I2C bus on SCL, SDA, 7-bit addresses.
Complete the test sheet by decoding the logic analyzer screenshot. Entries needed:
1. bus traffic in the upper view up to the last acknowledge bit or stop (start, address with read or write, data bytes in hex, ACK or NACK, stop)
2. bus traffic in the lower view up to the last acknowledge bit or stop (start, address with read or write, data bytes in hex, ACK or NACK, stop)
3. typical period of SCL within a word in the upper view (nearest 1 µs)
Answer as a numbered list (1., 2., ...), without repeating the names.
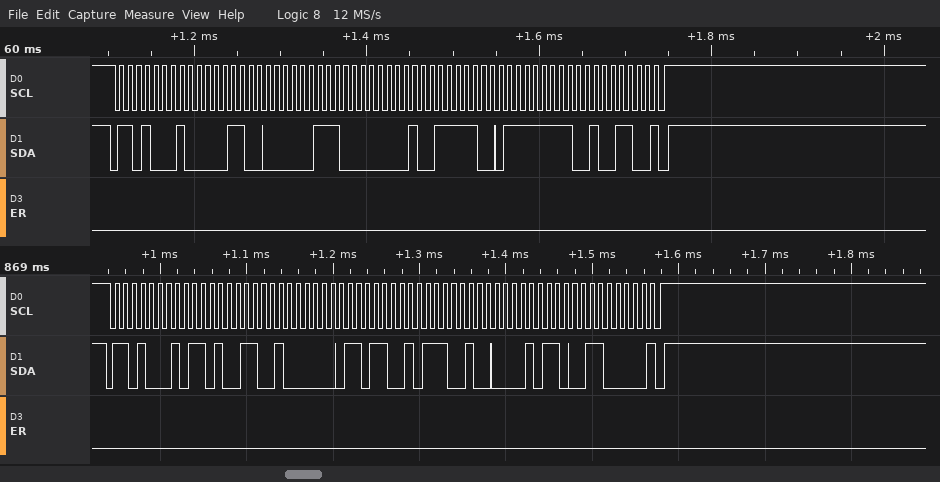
1. start, address 68 read ACK, 0C ACK, 07 ACK, 01 ACK, 7C ACK, FF ACK, 4C NACK, stop
2. start, address 68 read ACK, D3 ACK, 40 ACK, D9 ACK, E4 ACK, 16 ACK, 60 NACK, stop
3. 10 µs
